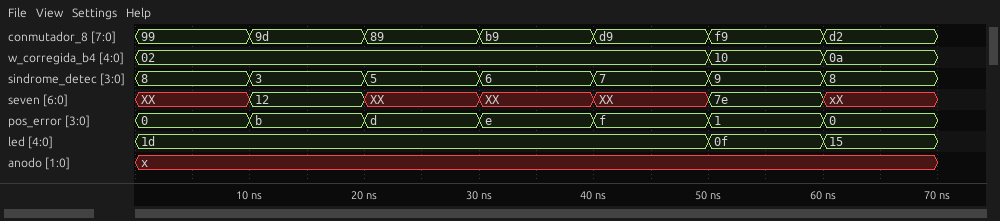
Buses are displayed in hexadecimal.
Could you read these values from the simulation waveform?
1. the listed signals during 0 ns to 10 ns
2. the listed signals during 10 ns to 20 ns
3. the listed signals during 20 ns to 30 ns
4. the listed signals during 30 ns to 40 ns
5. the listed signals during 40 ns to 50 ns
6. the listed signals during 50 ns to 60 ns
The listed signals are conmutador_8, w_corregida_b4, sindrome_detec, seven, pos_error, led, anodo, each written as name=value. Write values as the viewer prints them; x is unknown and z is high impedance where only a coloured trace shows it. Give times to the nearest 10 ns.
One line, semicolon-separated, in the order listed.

conmutador_8=99, w_corregida_b4=02, sindrome_detec=8, seven=XX, pos_error=0, led=1d, anodo=x; conmutador_8=9d, w_corregida_b4=02, sindrome_detec=3, seven=12, pos_error=b, led=1d, anodo=x; conmutador_8=89, w_corregida_b4=02, sindrome_detec=5, seven=XX, pos_error=d, led=1d, anodo=x; conmutador_8=b9, w_corregida_b4=02, sindrome_detec=6, seven=XX, pos_error=e, led=1d, anodo=x; conmutador_8=d9, w_corregida_b4=02, sindrome_detec=7, seven=XX, pos_error=f, led=1d, anodo=x; conmutador_8=f9, w_corregida_b4=10, sindrome_detec=9, seven=7e, pos_error=1, led=0f, anodo=x
